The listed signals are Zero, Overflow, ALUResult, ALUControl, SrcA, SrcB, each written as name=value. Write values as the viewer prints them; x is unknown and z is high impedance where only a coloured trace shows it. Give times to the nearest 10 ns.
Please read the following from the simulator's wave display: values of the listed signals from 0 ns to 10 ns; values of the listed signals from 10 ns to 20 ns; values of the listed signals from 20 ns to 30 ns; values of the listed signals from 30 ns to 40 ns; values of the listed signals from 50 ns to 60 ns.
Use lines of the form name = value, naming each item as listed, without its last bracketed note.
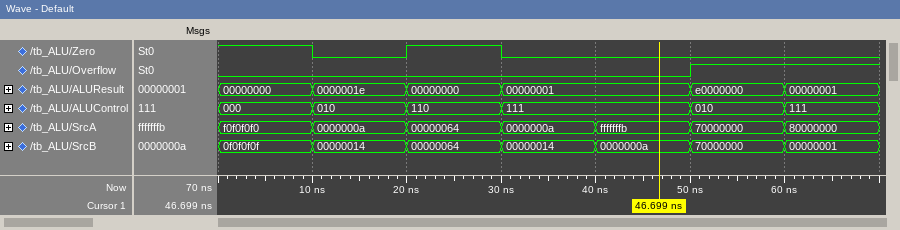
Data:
values of the listed signals from 0 ns to 10 ns = Zero=1, Overflow=0, ALUResult=00000000, ALUControl=000, SrcA=f0f0f0f0, SrcB=0f0f0f0f
values of the listed signals from 10 ns to 20 ns = Zero=0, Overflow=0, ALUResult=0000001e, ALUControl=010, SrcA=0000000a, SrcB=00000014
values of the listed signals from 20 ns to 30 ns = Zero=1, Overflow=0, ALUResult=00000000, ALUControl=110, SrcA=00000064, SrcB=00000064
values of the listed signals from 30 ns to 40 ns = Zero=0, Overflow=0, ALUResult=00000001, ALUControl=111, SrcA=0000000a, SrcB=00000014
values of the listed signals from 50 ns to 60 ns = Zero=0, Overflow=1, ALUResult=e0000000, ALUControl=010, SrcA=70000000, SrcB=70000000
